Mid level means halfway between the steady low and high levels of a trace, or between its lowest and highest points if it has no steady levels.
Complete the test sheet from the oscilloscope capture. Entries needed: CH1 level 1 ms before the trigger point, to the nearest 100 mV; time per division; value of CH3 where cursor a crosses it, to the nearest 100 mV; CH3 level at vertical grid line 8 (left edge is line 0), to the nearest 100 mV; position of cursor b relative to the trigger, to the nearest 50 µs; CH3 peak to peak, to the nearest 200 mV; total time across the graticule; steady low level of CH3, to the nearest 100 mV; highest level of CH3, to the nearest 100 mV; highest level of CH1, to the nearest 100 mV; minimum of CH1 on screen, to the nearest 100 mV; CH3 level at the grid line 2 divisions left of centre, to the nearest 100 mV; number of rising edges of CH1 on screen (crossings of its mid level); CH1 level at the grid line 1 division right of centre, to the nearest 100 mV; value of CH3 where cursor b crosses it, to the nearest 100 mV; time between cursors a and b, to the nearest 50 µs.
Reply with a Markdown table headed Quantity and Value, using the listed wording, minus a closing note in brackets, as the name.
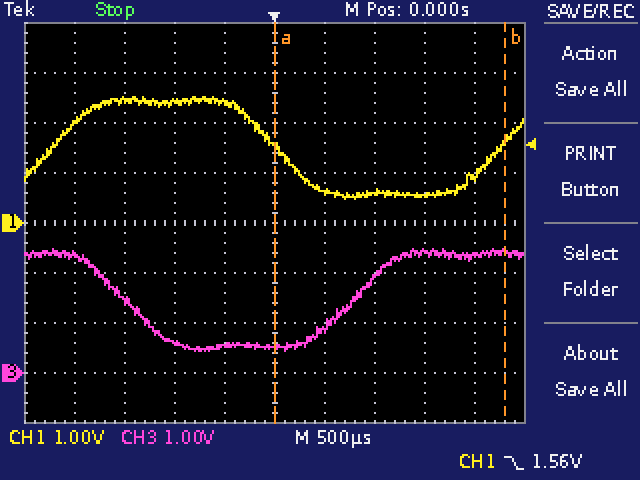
| Quantity | Value |
|---|---|
| CH1 level 1 ms before the trigger point, to the nearest 100 mV | 2.4 V |
| time per division | 500 µs |
| value of CH3 where cursor a crosses it, to the nearest 100 mV | 500 mV |
| CH3 level at vertical grid line 8 (left edge is line 0), to the nearest 100 mV | 2.4 V |
| position of cursor b relative to the trigger, to the nearest 50 µs | +2.30 ms |
| CH3 peak to peak, to the nearest 200 mV | 2.0 V |
| total time across the graticule | 5 ms |
| steady low level of CH3, to the nearest 100 mV | 500 mV |
| highest level of CH3, to the nearest 100 mV | 2.5 V |
| highest level of CH1, to the nearest 100 mV | 2.5 V |
| minimum of CH1 on screen, to the nearest 100 mV | 500 mV |
| CH3 level at the grid line 2 divisions left of centre, to the nearest 100 mV | 600 mV |
| number of rising edges of CH1 on screen | 2 |
| CH1 level at the grid line 1 division right of centre, to the nearest 100 mV | 600 mV |
| value of CH3 where cursor b crosses it, to the nearest 100 mV | 2.4 V |
| time between cursors a and b, to the nearest 50 µs | 2.30 ms |
